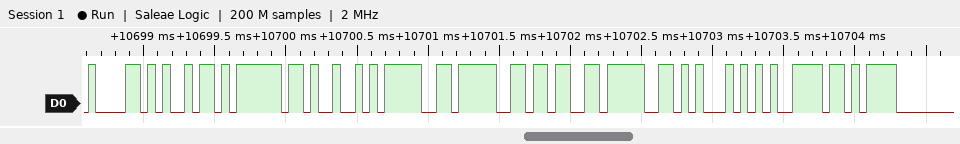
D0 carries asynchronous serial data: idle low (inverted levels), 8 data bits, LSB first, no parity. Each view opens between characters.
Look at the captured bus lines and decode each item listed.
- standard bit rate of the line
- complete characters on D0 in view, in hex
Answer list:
19200 baud
4F, 4B, 20, 5B, 30, 30, 32, 30, 5D, 0D, 0A
